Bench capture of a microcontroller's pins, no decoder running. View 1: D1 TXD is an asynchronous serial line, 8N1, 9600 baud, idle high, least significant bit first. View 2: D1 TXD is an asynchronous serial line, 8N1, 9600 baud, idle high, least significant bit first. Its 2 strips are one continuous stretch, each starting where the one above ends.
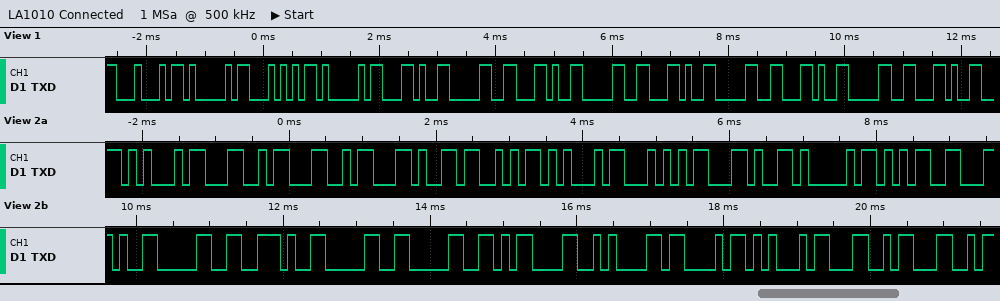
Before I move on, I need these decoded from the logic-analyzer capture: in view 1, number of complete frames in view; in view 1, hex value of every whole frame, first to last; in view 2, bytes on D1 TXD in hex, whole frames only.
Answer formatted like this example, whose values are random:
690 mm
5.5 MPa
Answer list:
13
44 41 54 41 2C 30 2C 30 2C 30 2C 30 2C
45 4C 4C 2C 53 45 54 2C 41 35 2C 30 2E 30 30 0D 0A 43 45 4C 4C
